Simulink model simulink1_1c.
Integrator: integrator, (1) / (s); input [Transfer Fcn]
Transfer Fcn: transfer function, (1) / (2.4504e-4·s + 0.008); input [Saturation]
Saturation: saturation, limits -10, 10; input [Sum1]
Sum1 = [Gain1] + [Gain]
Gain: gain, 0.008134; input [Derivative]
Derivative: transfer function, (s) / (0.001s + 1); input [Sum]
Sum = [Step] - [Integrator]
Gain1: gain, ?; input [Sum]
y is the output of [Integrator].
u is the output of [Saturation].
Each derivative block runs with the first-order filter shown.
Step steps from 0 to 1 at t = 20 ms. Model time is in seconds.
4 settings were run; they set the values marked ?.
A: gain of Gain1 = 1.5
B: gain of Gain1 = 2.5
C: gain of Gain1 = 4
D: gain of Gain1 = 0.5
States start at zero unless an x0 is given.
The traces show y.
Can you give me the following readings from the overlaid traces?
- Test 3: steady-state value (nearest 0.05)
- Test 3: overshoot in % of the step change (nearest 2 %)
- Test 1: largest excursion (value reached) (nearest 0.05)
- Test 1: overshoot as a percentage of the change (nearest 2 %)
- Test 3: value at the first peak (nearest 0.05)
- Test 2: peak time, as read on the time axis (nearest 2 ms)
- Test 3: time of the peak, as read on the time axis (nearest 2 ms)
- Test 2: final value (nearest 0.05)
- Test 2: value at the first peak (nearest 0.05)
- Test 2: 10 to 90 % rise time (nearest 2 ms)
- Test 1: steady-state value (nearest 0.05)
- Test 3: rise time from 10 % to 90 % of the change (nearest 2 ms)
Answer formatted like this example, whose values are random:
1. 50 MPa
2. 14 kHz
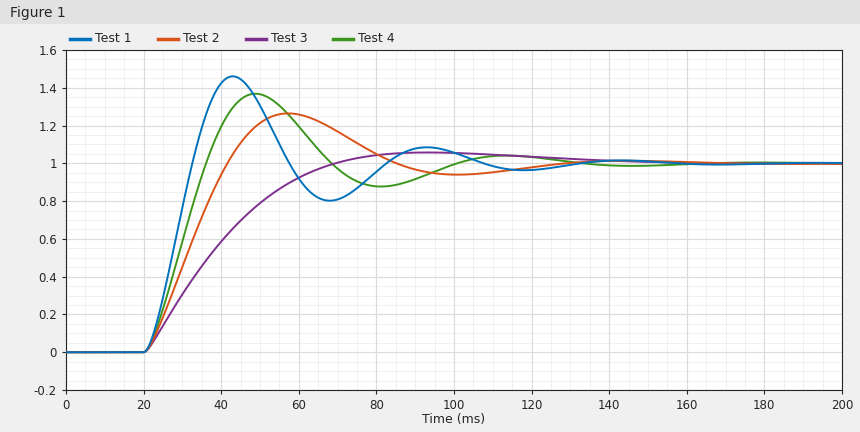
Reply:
1. 1.00
2. 6 %
3. 1.45
4. 46 %
5. 1.05
6. 58 ms
7. 94 ms
8. 1.00
9. 1.25
10. 16 ms
11. 1.00
12. 34 ms
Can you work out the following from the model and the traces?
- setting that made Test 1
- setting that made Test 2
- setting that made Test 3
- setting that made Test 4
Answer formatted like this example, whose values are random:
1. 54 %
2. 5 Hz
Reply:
1. C
2. A
3. D
4. B
